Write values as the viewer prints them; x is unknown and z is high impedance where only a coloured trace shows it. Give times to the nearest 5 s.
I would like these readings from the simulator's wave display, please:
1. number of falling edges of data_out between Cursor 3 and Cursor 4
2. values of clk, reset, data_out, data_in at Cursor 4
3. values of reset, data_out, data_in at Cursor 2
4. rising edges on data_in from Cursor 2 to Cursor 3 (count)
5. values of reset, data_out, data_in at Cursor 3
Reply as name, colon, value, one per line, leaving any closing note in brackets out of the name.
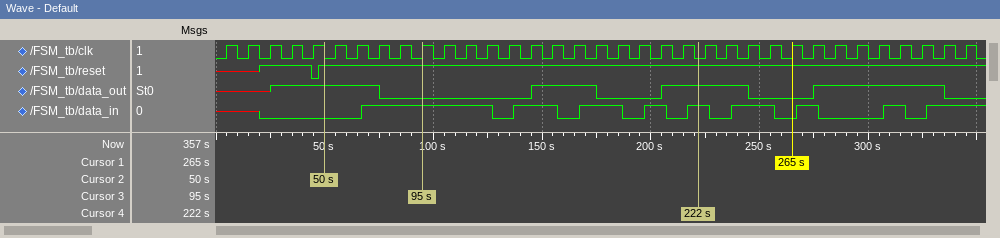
number of falling edges of data_out between Cursor 3 and Cursor 4: 1
values of clk, reset, data_out, data_in at Cursor 4: clk=0, reset=1, data_out=1, data_in=1
values of reset, data_out, data_in at Cursor 2: reset=1, data_out=1, data_in=0
rising edges on data_in from Cursor 2 to Cursor 3: 1
values of reset, data_out, data_in at Cursor 3: reset=1, data_out=0, data_in=1
